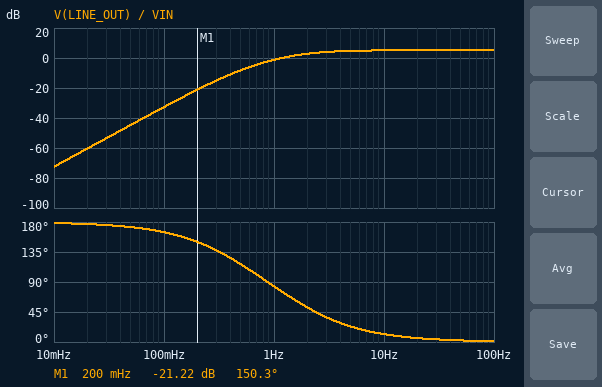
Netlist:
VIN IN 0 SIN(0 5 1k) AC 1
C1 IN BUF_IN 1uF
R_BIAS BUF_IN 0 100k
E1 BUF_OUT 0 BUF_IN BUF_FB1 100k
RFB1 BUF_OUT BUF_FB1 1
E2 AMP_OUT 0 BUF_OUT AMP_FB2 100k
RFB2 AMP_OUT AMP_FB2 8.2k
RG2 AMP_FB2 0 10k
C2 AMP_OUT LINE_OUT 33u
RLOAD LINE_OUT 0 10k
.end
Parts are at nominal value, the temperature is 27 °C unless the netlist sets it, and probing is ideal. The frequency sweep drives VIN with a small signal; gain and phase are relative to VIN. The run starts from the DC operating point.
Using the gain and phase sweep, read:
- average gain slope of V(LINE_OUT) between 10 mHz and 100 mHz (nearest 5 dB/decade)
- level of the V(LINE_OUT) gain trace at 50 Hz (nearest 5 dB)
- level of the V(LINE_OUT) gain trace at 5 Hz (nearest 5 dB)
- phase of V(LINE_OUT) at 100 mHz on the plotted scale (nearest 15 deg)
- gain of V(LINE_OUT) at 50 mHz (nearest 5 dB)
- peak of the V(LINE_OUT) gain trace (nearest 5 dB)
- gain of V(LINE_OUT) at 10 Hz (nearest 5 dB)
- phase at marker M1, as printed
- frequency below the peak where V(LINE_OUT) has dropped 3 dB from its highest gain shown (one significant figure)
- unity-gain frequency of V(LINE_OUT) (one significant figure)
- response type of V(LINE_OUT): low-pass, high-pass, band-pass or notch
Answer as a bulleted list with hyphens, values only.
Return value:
- 40 dB/decade
- 5 dB
- 5 dB
- 165 deg
- -45 dB
- 5 dB
- 5 dB
- 150.3 deg
- 2 Hz
- 1 Hz
- high-pass
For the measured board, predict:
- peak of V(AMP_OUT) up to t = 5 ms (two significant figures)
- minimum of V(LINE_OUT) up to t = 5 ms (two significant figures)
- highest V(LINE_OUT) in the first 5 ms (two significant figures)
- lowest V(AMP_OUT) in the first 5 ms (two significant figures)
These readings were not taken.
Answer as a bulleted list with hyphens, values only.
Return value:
- 9.1 V
- -9.1 V
- 9.1 V
- -9.1 V
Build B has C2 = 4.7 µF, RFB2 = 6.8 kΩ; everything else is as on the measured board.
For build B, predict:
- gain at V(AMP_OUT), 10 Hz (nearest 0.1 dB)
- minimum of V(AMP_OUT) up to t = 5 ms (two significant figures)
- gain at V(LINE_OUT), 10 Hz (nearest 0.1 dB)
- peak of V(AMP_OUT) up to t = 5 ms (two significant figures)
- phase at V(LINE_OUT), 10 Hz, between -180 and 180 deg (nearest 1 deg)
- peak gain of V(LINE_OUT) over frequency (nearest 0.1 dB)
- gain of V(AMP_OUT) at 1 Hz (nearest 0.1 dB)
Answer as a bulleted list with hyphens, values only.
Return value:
- 4.4 dB
- -8.4 V
- 3.9 dB
- 8.4 V
- 28 deg
- 4.5 dB
- -1.0 dB
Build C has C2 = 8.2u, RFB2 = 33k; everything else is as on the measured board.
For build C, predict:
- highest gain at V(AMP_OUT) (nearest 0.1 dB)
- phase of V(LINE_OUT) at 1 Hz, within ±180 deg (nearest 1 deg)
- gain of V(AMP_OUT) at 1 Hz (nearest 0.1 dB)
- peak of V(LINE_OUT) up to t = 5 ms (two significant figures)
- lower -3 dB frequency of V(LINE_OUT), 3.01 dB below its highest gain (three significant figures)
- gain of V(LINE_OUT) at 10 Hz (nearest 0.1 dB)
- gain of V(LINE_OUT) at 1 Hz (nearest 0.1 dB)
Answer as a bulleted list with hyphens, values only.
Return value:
- 12.7 dB
- 121 deg
- 7.2 dB
- 21 V
- 2.75 Hz
- 12.4 dB
- 0.4 dB
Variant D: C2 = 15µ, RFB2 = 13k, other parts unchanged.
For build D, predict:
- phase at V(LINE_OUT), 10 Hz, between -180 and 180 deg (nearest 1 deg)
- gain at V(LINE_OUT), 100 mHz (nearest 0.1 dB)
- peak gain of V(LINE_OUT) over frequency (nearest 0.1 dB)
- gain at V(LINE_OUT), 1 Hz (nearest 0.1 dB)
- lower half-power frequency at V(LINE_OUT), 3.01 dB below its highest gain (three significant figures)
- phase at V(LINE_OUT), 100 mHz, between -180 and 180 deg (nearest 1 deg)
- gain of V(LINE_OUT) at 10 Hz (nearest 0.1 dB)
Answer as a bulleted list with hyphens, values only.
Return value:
- 15 deg
- -37.4 dB
- 7.2 dB
- -1.5 dB
- 2.08 Hz
- 171 deg
- 7.1 dB
